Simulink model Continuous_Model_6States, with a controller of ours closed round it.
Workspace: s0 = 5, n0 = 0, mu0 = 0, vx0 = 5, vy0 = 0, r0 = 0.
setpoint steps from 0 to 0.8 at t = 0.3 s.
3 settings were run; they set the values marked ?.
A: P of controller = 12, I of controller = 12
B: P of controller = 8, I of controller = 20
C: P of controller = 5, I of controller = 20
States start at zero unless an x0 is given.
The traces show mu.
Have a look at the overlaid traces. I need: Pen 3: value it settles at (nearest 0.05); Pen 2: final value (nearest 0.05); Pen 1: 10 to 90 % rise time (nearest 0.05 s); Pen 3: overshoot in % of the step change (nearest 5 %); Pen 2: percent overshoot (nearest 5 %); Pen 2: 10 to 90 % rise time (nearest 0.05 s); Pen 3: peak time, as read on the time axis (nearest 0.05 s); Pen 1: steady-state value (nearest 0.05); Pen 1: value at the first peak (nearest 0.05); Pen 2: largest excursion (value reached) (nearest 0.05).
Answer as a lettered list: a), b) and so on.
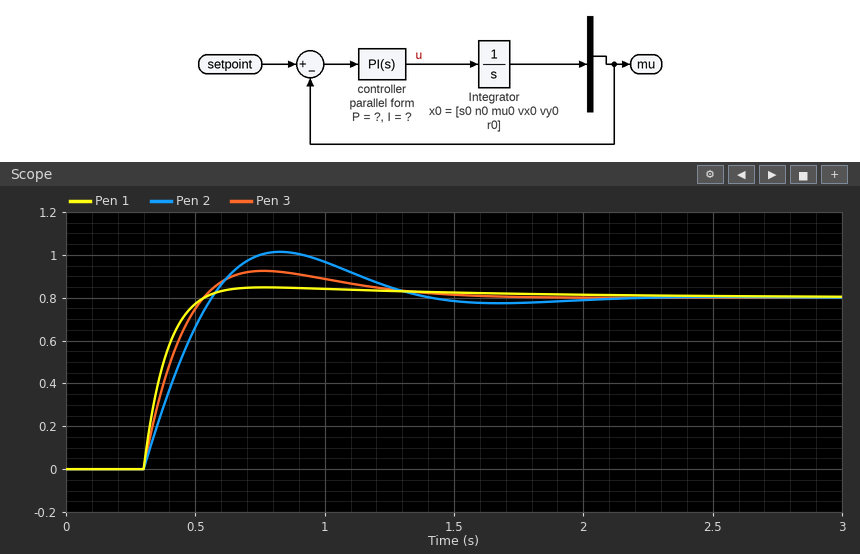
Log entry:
a) 0.80
b) 0.80
c) 0.15 s
d) 15 %
e) 25 %
f) 0.20 s
g) 0.75 s
h) 0.80
i) 0.85
j) 1.00
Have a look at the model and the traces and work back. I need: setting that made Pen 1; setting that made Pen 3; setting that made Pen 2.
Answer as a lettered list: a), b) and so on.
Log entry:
a) A
b) B
c) C
